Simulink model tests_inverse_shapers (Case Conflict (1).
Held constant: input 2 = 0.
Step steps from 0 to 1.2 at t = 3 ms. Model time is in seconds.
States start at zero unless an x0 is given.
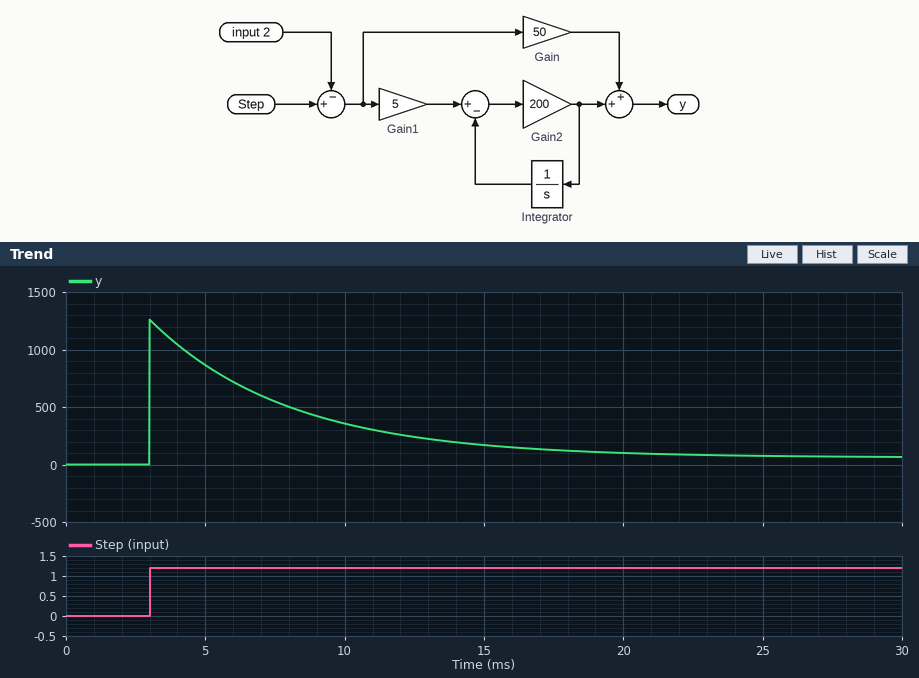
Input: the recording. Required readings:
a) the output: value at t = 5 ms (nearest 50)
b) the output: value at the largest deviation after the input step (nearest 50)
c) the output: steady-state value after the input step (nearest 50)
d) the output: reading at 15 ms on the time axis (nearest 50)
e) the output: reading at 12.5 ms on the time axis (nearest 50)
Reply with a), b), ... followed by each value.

a) 850
b) 1250
c) 50
d) 150
e) 250
